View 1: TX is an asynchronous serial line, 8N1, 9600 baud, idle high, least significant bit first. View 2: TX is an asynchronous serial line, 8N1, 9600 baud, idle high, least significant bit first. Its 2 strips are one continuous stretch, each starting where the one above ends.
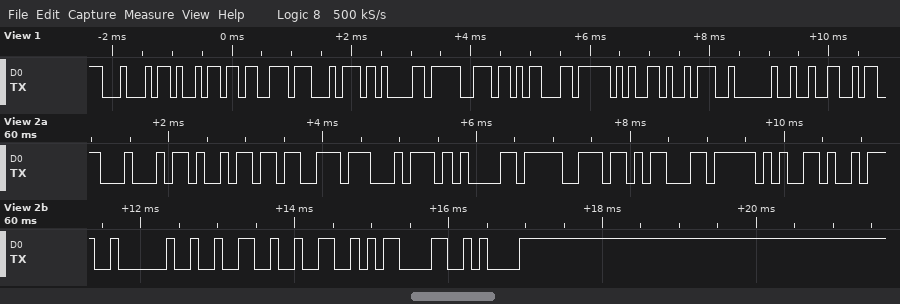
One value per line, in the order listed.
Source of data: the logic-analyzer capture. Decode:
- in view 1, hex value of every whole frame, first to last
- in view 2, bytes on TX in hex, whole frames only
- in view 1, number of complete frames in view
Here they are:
44 69 73 74 61 6E 63 65 3A 20 32
0x44 0x69 0x73 0x74 0x61 0x6E 0x63 0x65 0x3A 0x20 0x32 0x32 0x0D 0x0A
11
